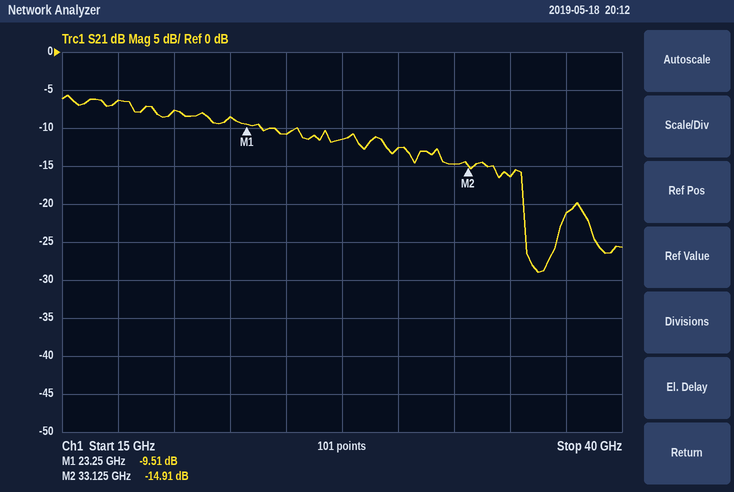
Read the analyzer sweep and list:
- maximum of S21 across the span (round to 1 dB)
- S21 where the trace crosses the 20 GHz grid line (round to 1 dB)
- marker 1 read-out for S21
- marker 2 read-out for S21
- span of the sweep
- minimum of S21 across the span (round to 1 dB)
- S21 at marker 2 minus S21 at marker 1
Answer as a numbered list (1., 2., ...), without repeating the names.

1. -6 dB
2. -8 dB
3. -9.51 dB
4. -14.91 dB
5. 25 GHz
6. -29 dB
7. -5.40 dB
